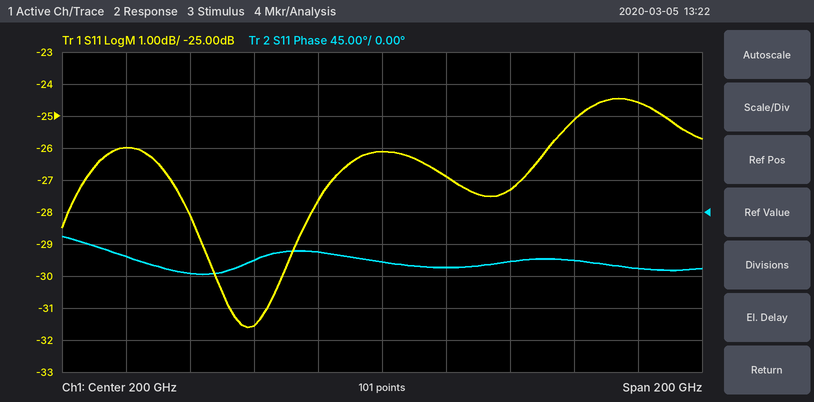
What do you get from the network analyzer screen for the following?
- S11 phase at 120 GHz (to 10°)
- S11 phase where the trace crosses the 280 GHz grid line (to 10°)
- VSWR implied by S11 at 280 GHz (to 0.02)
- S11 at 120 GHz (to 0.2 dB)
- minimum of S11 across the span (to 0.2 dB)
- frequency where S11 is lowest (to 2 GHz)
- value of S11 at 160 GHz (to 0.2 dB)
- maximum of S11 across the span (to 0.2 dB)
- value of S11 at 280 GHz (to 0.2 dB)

-60°
-80°
1.12
-26.0 dB
-31.6 dB
158 GHz
-31.6 dB
-24.4 dB
-24.6 dB
